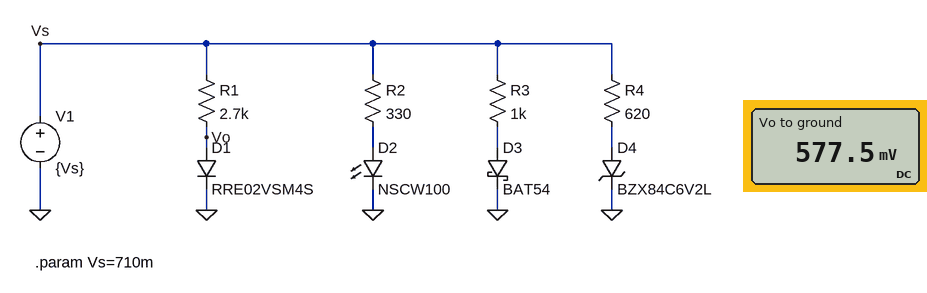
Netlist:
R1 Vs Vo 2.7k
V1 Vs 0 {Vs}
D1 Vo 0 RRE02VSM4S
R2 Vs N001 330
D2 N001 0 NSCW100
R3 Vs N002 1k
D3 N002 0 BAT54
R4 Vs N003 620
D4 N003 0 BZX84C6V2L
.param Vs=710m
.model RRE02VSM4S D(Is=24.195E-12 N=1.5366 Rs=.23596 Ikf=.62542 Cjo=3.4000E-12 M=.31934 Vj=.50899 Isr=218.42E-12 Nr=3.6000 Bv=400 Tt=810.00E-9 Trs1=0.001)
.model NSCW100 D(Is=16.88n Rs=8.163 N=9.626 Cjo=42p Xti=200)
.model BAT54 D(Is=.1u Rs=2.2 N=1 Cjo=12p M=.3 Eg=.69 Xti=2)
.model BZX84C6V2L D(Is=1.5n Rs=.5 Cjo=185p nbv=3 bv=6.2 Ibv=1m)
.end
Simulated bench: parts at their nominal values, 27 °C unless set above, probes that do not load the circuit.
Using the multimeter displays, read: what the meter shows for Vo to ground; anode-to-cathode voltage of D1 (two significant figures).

577.5 mV
580 mV
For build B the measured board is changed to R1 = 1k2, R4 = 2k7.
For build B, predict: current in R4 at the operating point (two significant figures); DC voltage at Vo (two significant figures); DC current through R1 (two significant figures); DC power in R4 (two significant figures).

150 µA
600 mV
90 µA
63 µW
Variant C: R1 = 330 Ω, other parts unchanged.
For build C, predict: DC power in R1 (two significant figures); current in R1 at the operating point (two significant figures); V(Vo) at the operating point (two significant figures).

16 µW
220 µA
640 mV
